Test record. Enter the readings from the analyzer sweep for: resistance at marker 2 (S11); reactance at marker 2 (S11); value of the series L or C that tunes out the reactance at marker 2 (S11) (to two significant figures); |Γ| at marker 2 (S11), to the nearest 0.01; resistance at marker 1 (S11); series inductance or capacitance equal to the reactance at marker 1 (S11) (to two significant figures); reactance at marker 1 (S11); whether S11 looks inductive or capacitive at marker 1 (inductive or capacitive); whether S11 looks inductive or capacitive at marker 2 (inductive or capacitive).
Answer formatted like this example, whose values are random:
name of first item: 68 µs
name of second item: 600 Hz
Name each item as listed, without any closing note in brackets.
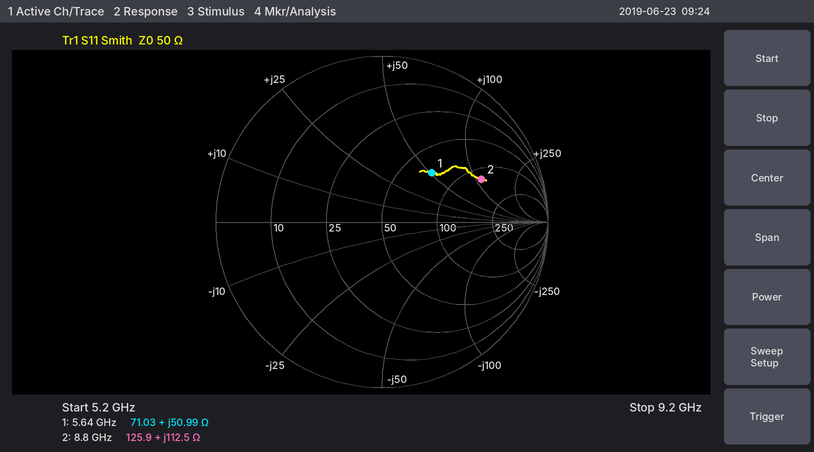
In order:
resistance at marker 2: 125.9 Ω
reactance at marker 2: +112.5 Ω
value of the series L or C that tunes out the reactance at marker 2 (S11): 160 fF
|Γ| at marker 2 (S11), to the nearest 0.01: 0.65
resistance at marker 1: 71.03 Ω
series inductance or capacitance equal to the reactance at marker 1 (S11): 1.4 nH
reactance at marker 1: +50.99 Ω
whether S11 looks inductive or capacitive at marker 1: inductive
whether S11 looks inductive or capacitive at marker 2: inductive
